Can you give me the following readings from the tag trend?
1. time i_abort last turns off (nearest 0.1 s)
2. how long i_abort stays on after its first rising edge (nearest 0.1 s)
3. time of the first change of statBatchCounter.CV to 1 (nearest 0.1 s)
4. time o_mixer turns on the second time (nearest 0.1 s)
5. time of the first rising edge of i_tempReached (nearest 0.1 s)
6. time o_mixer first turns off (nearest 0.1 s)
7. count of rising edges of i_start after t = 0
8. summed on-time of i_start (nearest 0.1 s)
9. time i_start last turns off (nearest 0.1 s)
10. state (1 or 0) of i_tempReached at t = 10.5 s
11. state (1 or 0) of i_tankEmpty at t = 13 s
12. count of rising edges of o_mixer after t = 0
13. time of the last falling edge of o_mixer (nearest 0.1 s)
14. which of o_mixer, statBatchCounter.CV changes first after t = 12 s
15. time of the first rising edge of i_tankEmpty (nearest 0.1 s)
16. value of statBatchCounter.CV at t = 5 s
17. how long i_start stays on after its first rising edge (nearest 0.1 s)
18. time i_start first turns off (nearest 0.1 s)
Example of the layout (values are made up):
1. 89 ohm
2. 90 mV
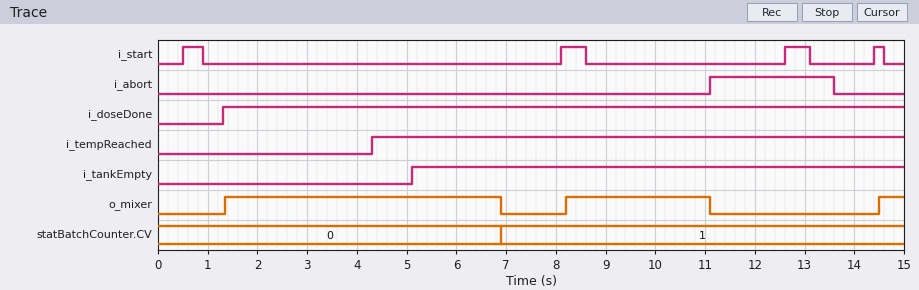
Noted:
1. 13.6 s
2. 2.5 s
3. 6.9 s
4. 8.2 s
5. 4.3 s
6. 6.9 s
7. 4
8. 1.6 s
9. 14.6 s
10. 1
11. 1
12. 3
13. 11.1 s
14. o_mixer
15. 5.1 s
16. 0
17. 0.4 s
18. 0.9 s
